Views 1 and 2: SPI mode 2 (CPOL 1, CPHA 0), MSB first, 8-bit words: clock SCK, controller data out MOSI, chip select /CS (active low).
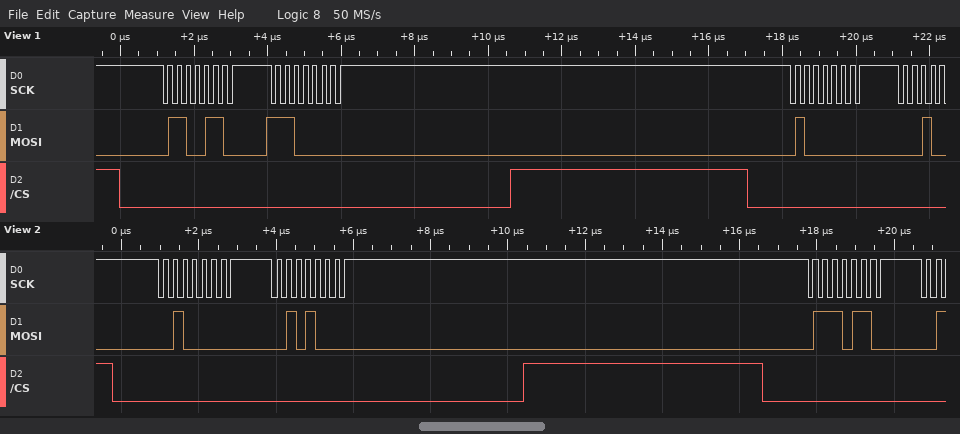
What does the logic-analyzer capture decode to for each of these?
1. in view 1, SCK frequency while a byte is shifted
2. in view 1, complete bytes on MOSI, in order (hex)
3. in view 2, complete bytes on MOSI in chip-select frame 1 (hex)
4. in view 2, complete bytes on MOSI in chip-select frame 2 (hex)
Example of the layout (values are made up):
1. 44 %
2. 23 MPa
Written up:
1. 4 MHz
2. 66 E0 40
3. 20 28
4. 76
